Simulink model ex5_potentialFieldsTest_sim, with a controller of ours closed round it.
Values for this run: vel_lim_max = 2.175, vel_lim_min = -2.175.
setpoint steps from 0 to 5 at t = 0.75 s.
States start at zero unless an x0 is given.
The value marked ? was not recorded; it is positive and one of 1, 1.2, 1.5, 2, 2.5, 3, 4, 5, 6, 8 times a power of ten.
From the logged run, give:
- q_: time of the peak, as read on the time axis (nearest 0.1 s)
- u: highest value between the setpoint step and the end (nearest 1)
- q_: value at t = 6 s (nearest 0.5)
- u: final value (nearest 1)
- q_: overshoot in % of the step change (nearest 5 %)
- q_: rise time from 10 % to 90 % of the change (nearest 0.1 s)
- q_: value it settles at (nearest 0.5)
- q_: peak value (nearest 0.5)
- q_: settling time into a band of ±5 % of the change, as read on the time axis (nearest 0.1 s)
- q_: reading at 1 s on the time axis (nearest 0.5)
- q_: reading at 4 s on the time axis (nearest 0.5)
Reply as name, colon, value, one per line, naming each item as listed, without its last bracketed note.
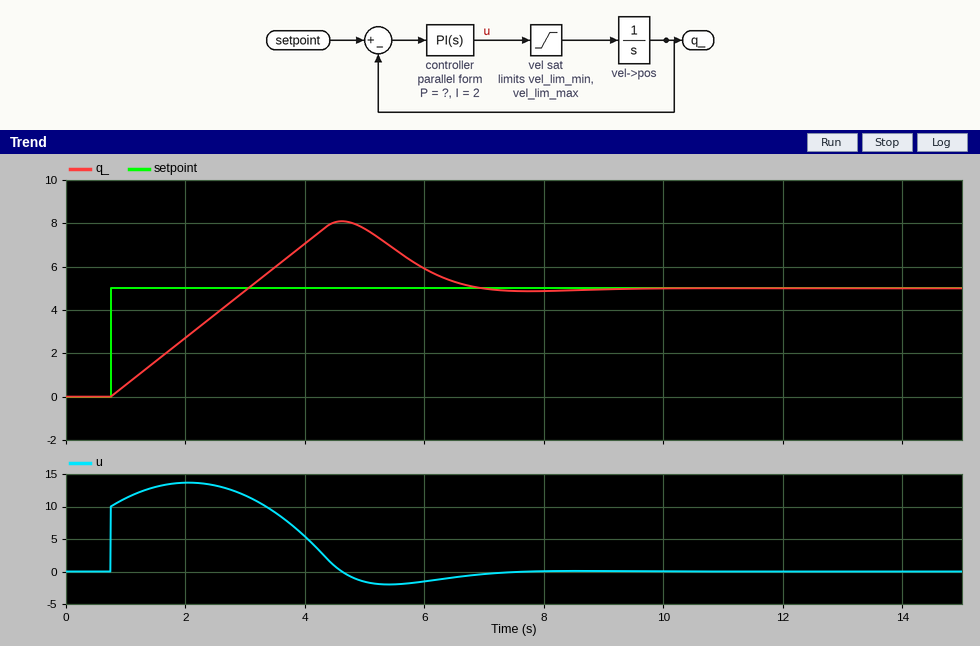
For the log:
q_: time of the peak, as read on the time axis: 4.6 s
u: highest value between the setpoint step and the end: 14
q_: value at t = 6 s: 6.0
u: final value: 0
q_: overshoot in % of the step change: 60 %
q_: rise time from 10 % to 90 % of the change: 1.8 s
q_: value it settles at: 5.0
q_: peak value: 8.0
q_: settling time into a band of ±5 % of the change, as read on the time axis: 6.6 s
q_: reading at 1 s on the time axis: 0.5
q_: reading at 4 s on the time axis: 7.0
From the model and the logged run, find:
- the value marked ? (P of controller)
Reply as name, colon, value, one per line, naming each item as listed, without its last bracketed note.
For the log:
the value marked ?: 2
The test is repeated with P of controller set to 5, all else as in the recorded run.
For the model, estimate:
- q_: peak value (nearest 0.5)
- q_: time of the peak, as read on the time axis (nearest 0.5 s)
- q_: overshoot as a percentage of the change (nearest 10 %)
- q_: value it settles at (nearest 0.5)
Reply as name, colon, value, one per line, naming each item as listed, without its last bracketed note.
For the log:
q_: peak value: 7.0
q_: time of the peak, as read on the time axis: 4.0 s
q_: overshoot as a percentage of the change: 40 %
q_: value it settles at: 5.0
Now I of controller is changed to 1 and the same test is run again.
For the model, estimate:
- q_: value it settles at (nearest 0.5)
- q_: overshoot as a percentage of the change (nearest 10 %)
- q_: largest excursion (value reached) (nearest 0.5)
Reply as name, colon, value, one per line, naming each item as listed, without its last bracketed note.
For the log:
q_: value it settles at: 5.0
q_: overshoot as a percentage of the change: 40 %
q_: largest excursion (value reached): 7.0
